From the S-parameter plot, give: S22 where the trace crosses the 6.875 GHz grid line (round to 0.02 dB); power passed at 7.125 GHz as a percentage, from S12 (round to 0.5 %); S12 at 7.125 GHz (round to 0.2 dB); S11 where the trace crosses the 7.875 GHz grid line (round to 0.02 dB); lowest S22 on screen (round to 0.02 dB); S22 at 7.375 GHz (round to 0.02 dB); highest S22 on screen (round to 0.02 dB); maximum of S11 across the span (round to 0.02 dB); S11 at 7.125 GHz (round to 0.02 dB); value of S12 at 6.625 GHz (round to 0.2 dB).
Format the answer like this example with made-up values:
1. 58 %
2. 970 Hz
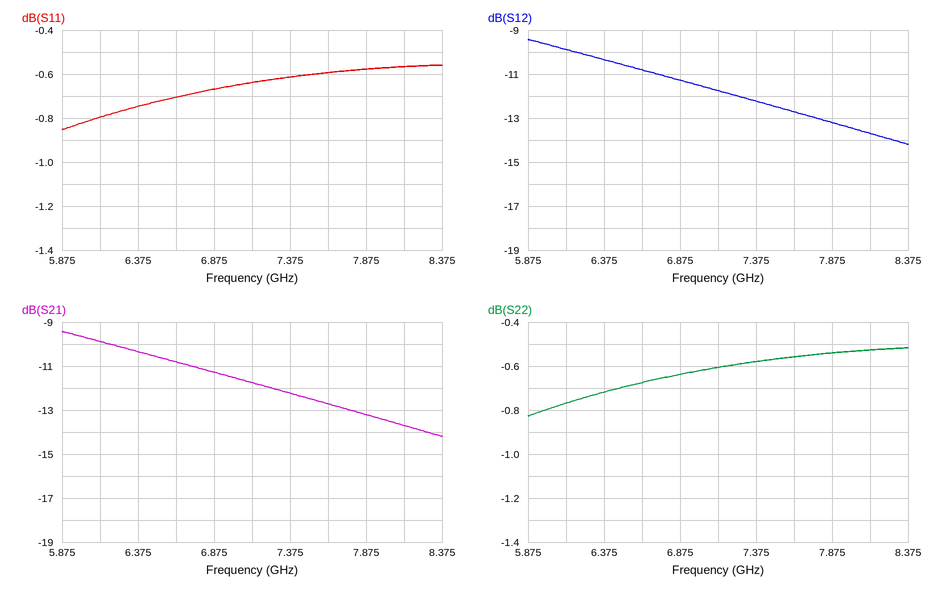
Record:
1. -0.64 dB
2. 6.5 %
3. -11.8 dB
4. -0.58 dB
5. -0.82 dB
6. -0.58 dB
7. -0.52 dB
8. -0.56 dB
9. -0.64 dB
10. -10.8 dB
